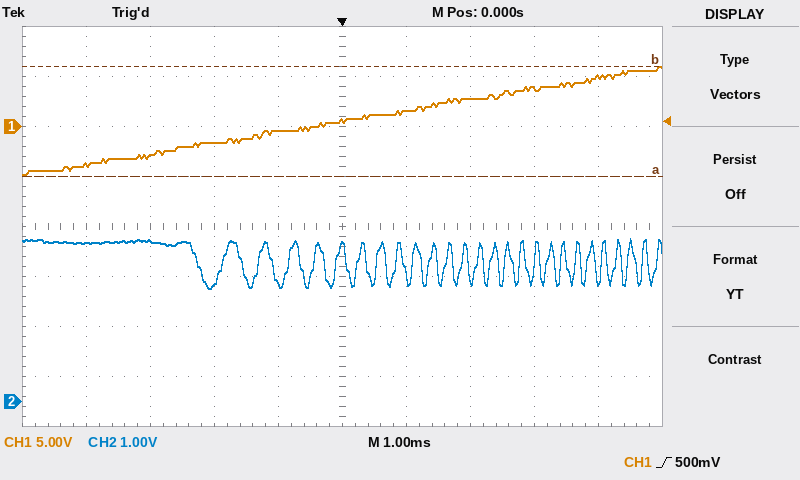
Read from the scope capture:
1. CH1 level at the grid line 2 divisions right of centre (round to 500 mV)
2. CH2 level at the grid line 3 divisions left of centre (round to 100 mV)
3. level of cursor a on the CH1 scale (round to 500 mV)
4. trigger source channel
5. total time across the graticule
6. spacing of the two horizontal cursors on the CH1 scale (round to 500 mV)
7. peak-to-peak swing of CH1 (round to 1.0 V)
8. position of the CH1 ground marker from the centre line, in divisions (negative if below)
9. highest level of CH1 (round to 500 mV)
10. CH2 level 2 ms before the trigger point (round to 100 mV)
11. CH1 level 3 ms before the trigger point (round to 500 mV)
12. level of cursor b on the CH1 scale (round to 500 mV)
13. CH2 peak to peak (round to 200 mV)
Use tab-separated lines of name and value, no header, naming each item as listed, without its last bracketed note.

CH1 level at the grid line 2 divisions right of centre	3.0 V
CH2 level at the grid line 3 divisions left of centre	3.2 V
level of cursor a on the CH1 scale	-5.0 V
trigger source channel	CH1
total time across the graticule	10 ms
spacing of the two horizontal cursors on the CH1 scale	11.0 V
peak-to-peak swing of CH1	11.0 V
position of the CH1 ground marker from the centre line, in divisions	+2.0 div
highest level of CH1	6.0 V
CH2 level 2 ms before the trigger point	2.4 V
CH1 level 3 ms before the trigger point	-3.0 V
level of cursor b on the CH1 scale	6.0 V
CH2 peak to peak	1.0 V
